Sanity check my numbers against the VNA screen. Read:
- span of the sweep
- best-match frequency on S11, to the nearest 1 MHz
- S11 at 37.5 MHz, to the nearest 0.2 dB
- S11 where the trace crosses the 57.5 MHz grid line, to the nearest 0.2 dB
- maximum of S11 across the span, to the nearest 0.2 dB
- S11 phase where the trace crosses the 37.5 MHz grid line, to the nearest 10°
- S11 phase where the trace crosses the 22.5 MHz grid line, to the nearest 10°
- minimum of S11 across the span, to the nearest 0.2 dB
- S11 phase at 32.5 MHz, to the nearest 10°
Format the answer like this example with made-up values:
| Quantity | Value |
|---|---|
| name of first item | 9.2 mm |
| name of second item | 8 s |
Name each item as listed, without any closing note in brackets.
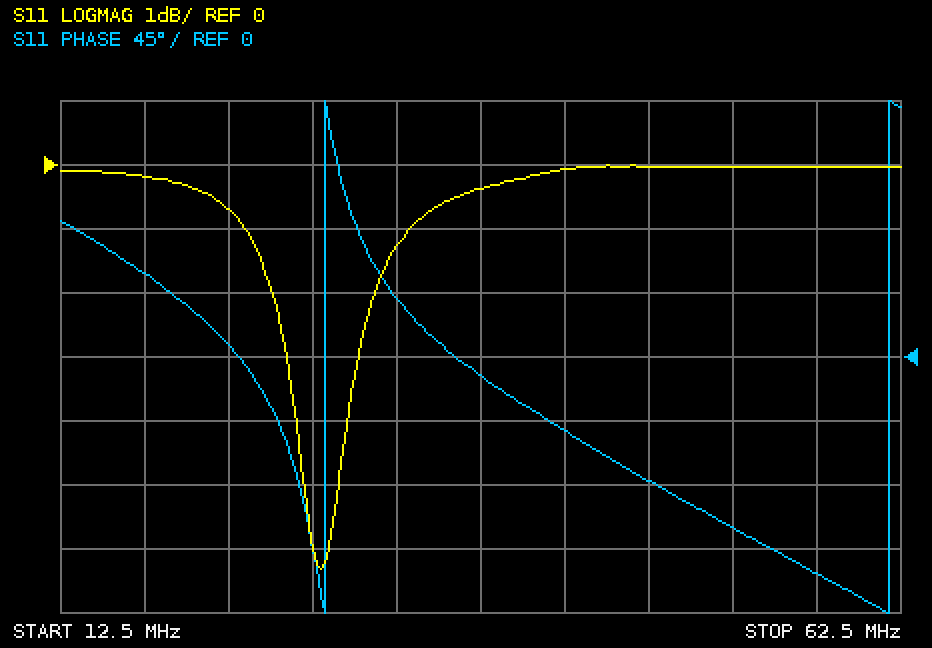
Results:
| Quantity | Value |
|---|---|
| span of the sweep | 50 MHz |
| best-match frequency on S11, to the nearest 1 MHz | 28 MHz |
| S11 at 37.5 MHz, to the nearest 0.2 dB | -0.4 dB |
| S11 where the trace crosses the 57.5 MHz grid line, to the nearest 0.2 dB | 0.0 dB |
| maximum of S11 across the span, to the nearest 0.2 dB | 0.0 dB |
| S11 phase where the trace crosses the 37.5 MHz grid line, to the nearest 10° | -10° |
| S11 phase where the trace crosses the 22.5 MHz grid line, to the nearest 10° | 10° |
| minimum of S11 across the span, to the nearest 0.2 dB | -6.4 dB |
| S11 phase at 32.5 MHz, to the nearest 10° | 40° |
